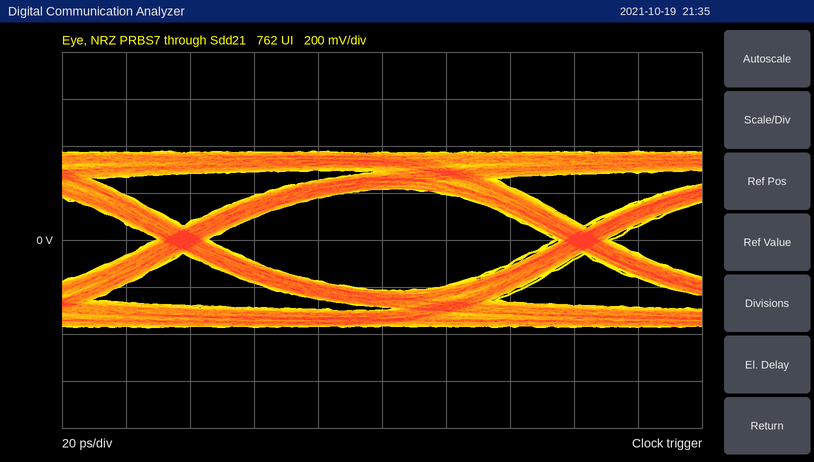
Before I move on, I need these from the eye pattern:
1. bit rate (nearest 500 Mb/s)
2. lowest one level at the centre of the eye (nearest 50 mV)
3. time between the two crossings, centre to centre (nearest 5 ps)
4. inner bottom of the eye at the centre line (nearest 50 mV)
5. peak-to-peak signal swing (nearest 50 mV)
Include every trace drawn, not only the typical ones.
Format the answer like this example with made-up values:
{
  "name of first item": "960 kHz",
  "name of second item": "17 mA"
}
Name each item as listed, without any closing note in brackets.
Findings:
{
  "bit rate": "8.0 Gb/s",
  "lowest one level at the centre of the eye": "200 mV",
  "time between the two crossings, centre to centre": "125 ps",
  "inner bottom of the eye at the centre line": "-200 mV",
  "peak-to-peak signal swing": "750 mV"
}
